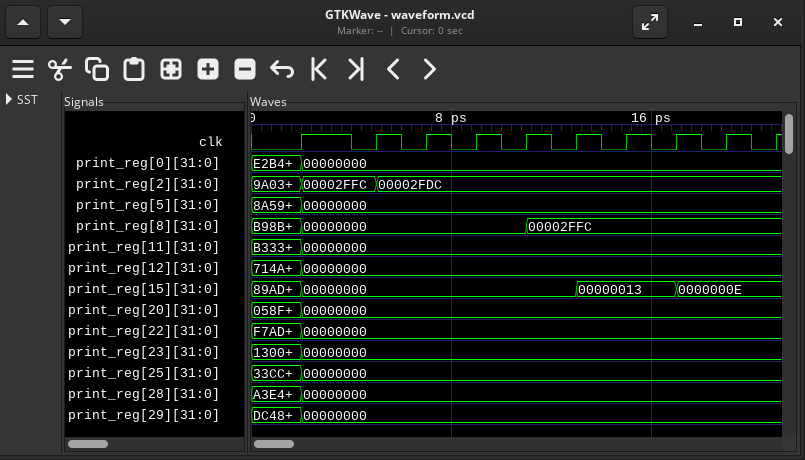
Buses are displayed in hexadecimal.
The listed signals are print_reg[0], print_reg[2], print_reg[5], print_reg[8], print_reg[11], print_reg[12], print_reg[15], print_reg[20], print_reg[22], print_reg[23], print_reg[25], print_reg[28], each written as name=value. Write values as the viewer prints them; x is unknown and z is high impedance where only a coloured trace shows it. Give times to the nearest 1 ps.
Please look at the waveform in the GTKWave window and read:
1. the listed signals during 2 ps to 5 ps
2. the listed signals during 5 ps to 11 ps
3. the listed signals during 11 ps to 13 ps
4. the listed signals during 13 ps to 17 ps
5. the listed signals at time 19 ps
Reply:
print_reg[0]=00000000, print_reg[2]=00002FFC, print_reg[5]=00000000, print_reg[8]=00000000, print_reg[11]=00000000, print_reg[12]=00000000, print_reg[15]=00000000, print_reg[20]=00000000, print_reg[22]=00000000, print_reg[23]=00000000, print_reg[25]=00000000, print_reg[28]=00000000
print_reg[0]=00000000, print_reg[2]=00002FDC, print_reg[5]=00000000, print_reg[8]=00000000, print_reg[11]=00000000, print_reg[12]=00000000, print_reg[15]=00000000, print_reg[20]=00000000, print_reg[22]=00000000, print_reg[23]=00000000, print_reg[25]=00000000, print_reg[28]=00000000
print_reg[0]=00000000, print_reg[2]=00002FDC, print_reg[5]=00000000, print_reg[8]=00002FFC, print_reg[11]=00000000, print_reg[12]=00000000, print_reg[15]=00000000, print_reg[20]=00000000, print_reg[22]=00000000, print_reg[23]=00000000, print_reg[25]=00000000, print_reg[28]=00000000
print_reg[0]=00000000, print_reg[2]=00002FDC, print_reg[5]=00000000, print_reg[8]=00002FFC, print_reg[11]=00000000, print_reg[12]=00000000, print_reg[15]=00000013, print_reg[20]=00000000, print_reg[22]=00000000, print_reg[23]=00000000, print_reg[25]=00000000, print_reg[28]=00000000
print_reg[0]=00000000, print_reg[2]=00002FDC, print_reg[5]=00000000, print_reg[8]=00002FFC, print_reg[11]=00000000, print_reg[12]=00000000, print_reg[15]=0000000E, print_reg[20]=00000000, print_reg[22]=00000000, print_reg[23]=00000000, print_reg[25]=00000000, print_reg[28]=00000000
